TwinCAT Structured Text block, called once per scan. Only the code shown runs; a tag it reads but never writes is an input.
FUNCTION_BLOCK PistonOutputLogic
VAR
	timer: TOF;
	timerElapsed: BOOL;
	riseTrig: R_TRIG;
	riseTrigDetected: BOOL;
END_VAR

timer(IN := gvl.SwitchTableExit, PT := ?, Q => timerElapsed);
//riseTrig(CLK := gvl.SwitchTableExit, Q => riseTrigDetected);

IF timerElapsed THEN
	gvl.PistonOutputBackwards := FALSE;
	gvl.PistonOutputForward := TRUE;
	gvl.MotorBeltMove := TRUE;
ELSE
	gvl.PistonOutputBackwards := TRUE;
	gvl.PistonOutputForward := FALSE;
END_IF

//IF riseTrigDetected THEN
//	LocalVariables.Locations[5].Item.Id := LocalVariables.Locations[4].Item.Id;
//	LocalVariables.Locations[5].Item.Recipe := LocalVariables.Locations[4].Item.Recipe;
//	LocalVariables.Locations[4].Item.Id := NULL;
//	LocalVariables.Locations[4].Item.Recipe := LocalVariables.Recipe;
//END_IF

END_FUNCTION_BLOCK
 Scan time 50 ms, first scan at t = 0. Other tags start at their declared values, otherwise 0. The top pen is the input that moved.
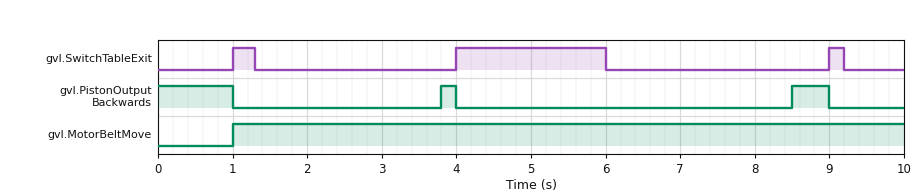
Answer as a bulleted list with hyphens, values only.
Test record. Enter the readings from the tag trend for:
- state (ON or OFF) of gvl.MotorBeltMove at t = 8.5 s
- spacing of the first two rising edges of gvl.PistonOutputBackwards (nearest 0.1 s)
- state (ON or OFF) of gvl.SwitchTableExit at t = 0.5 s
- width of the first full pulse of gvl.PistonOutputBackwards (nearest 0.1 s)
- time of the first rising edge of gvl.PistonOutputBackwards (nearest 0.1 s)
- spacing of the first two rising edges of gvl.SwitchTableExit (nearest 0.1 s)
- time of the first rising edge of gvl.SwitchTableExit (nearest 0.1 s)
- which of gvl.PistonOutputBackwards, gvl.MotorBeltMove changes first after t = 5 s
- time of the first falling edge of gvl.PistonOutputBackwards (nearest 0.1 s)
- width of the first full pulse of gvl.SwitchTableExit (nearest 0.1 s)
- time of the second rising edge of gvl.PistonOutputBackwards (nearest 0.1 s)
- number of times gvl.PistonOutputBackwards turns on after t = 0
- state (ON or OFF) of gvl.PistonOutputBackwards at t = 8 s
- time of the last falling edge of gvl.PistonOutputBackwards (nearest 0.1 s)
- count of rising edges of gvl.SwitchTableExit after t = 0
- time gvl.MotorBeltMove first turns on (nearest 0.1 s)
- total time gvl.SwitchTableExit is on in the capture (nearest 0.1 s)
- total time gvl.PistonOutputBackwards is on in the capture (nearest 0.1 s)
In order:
- ON
- 4.7 s
- OFF
- 0.2 s
- 3.8 s
- 3.0 s
- 1.0 s
- gvl.PistonOutputBackwards
- 1.0 s
- 0.3 s
- 8.5 s
- 2
- OFF
- 9.0 s
- 3
- 1.0 s
- 2.5 s
- 1.7 s
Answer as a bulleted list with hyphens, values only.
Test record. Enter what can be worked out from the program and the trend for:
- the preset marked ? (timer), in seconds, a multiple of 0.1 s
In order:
- 2.5 s
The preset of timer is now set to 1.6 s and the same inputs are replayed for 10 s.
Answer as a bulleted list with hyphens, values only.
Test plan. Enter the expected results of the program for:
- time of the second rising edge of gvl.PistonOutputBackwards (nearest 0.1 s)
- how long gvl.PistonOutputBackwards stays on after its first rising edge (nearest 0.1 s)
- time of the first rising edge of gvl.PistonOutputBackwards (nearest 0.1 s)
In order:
- 7.6 s
- 1.1 s
- 2.9 s
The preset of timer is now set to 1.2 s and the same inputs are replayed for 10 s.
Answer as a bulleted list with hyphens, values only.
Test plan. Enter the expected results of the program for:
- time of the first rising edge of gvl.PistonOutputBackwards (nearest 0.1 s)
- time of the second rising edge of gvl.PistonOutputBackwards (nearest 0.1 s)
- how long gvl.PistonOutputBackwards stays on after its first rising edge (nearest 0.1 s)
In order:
- 2.5 s
- 7.2 s
- 1.5 s
